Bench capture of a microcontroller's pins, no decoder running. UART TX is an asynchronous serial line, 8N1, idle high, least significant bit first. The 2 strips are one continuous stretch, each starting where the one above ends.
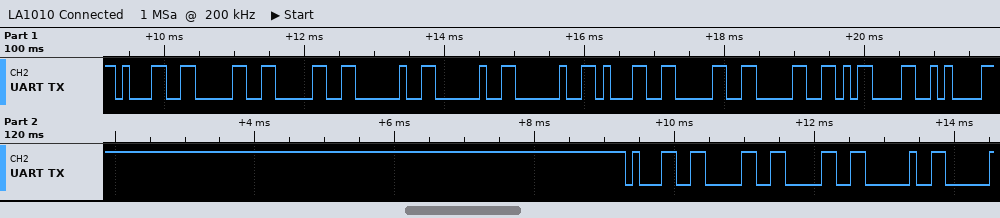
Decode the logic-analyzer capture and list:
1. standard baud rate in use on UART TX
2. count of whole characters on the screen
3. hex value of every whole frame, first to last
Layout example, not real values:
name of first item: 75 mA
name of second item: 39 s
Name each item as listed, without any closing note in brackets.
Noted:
standard baud rate in use on UART TX: 9600 baud
count of whole characters on the screen: 15
hex value of every whole frame, first to last: 0x31 0x30 0x30 0x20 0x20 0x20 0x31 0x30 0x30 0x0D 0x0A 0x31 0x30 0x30 0x20
